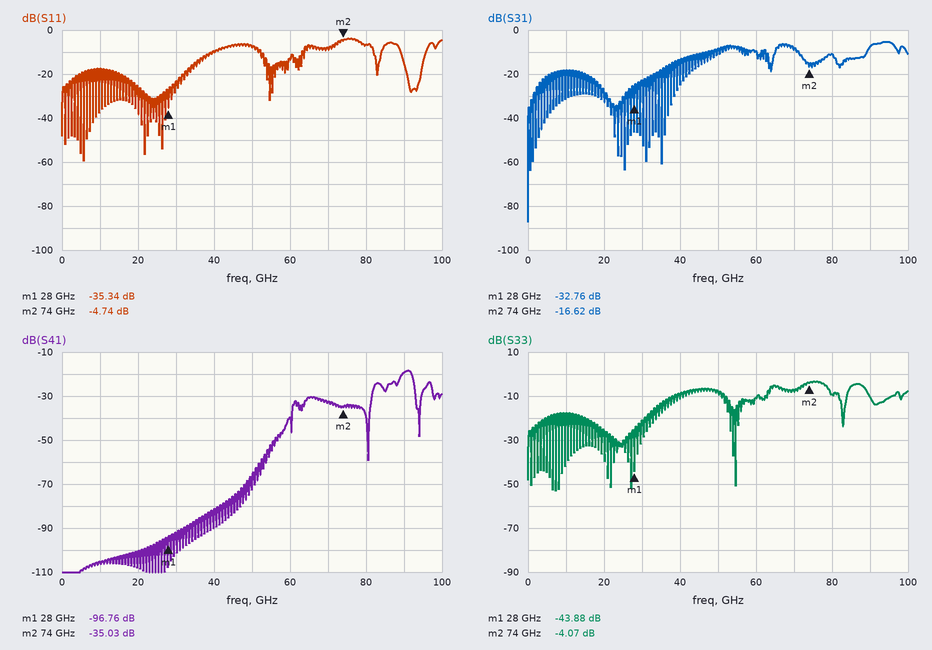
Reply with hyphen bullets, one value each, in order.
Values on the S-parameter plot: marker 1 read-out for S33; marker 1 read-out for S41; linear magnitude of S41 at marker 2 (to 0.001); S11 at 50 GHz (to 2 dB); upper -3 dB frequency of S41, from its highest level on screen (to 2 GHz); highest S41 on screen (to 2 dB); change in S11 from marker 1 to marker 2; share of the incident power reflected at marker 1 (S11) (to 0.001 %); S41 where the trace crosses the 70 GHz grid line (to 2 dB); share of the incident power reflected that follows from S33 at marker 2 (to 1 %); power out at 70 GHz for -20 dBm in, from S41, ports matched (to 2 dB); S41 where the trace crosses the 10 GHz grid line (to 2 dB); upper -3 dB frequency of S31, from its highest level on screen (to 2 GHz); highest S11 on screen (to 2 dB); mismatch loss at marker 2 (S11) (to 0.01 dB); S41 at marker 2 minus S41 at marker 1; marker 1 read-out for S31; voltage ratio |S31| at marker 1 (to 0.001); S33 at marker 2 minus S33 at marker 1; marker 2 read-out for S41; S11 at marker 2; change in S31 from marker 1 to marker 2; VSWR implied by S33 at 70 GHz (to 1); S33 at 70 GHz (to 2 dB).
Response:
- -43.88 dB
- -96.76 dB
- 0.018
- -8 dB
- 92 GHz
- -18 dB
- 30.60 dB
- 0.029 %
- -32 dB
- 39 %
- -52 dBm
- -106 dB
- 96 GHz
- -4 dB
- 1.78 dB
- 61.73 dB
- -32.76 dB
- 0.023
- 39.81 dB
- -35.03 dB
- -4.74 dB
- 16.14 dB
- 2
- -8 dB
